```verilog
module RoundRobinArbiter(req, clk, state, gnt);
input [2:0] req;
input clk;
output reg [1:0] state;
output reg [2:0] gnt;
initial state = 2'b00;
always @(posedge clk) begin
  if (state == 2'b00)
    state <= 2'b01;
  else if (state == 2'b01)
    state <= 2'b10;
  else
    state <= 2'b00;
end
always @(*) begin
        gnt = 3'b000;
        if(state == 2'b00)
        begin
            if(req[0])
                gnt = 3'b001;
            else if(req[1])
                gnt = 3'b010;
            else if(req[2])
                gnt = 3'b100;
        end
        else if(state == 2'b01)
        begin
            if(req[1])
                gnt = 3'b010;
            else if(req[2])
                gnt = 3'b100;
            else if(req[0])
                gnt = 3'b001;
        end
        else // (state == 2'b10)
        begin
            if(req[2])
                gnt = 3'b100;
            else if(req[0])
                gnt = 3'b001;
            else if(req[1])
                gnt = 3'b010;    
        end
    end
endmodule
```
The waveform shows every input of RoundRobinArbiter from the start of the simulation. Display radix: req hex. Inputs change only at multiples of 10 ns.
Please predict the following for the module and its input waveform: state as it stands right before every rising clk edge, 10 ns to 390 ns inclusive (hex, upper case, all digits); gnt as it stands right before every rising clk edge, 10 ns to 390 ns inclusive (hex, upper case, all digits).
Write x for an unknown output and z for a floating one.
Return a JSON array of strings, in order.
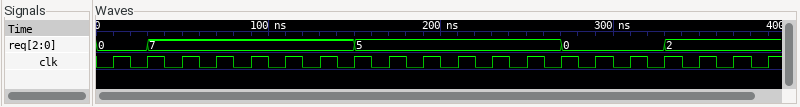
["0, 1, 2, 0, 1, 2, 0, 1, 2, 0, 1, 2, 0, 1, 2, 0, 1, 2, 0, 1", "0, 0, 4, 1, 2, 4, 1, 2, 4, 1, 4, 4, 1, 4, 0, 0, 0, 2, 2, 2"]
